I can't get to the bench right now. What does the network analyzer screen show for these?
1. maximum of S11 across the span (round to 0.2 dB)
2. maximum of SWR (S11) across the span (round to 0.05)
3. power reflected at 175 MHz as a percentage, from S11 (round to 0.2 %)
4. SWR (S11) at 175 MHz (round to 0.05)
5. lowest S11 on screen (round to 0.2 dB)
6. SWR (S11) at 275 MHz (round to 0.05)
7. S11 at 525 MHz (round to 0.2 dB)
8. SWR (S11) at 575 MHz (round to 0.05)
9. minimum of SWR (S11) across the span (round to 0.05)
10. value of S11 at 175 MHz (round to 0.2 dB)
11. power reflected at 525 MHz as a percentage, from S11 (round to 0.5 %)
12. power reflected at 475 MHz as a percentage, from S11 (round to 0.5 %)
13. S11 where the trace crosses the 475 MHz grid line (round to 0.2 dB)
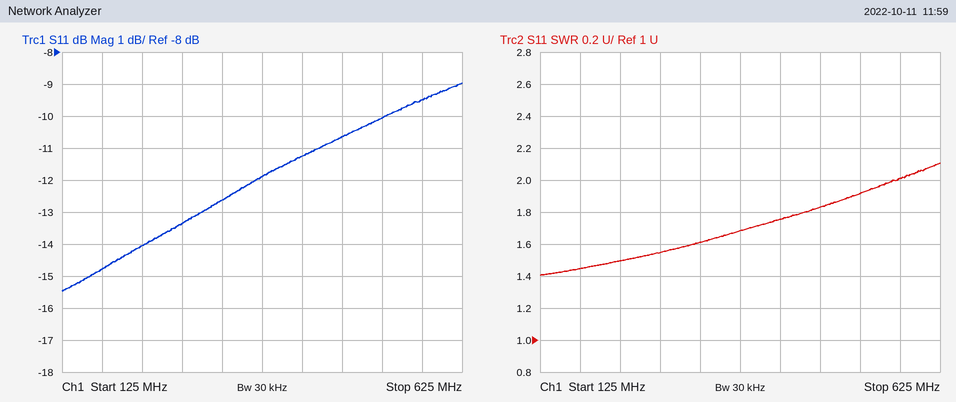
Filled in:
-9.0 dB
2.10
3.4 %
1.45
-15.4 dB
1.55
-10.0 dB
2.00
1.40
-14.8 dB
10.0 %
8.5 %
-10.6 dB
